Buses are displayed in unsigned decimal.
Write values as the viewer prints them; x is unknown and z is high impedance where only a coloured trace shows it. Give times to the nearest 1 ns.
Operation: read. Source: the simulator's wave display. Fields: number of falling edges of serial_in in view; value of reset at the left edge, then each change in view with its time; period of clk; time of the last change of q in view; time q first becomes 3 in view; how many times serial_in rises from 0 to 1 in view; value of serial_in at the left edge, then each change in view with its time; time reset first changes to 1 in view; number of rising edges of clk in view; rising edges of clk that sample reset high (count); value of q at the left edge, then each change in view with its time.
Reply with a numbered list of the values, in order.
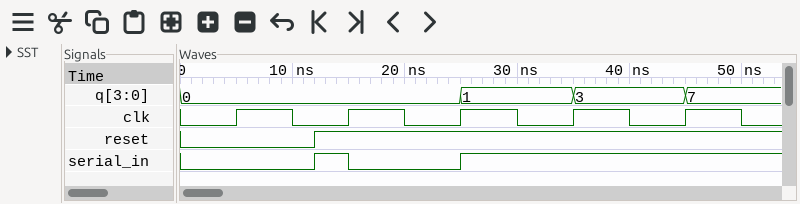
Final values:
1. 1
2. 0, 1 at 12 ns
3. 10 ns
4. 45 ns
5. 35 ns
6. 2
7. 0, 1 at 12 ns, 0 at 15 ns, 1 at 25 ns
8. 12 ns
9. 5
10. 4
11. 0, 1 at 25 ns, 3 at 35 ns, 7 at 45 ns
